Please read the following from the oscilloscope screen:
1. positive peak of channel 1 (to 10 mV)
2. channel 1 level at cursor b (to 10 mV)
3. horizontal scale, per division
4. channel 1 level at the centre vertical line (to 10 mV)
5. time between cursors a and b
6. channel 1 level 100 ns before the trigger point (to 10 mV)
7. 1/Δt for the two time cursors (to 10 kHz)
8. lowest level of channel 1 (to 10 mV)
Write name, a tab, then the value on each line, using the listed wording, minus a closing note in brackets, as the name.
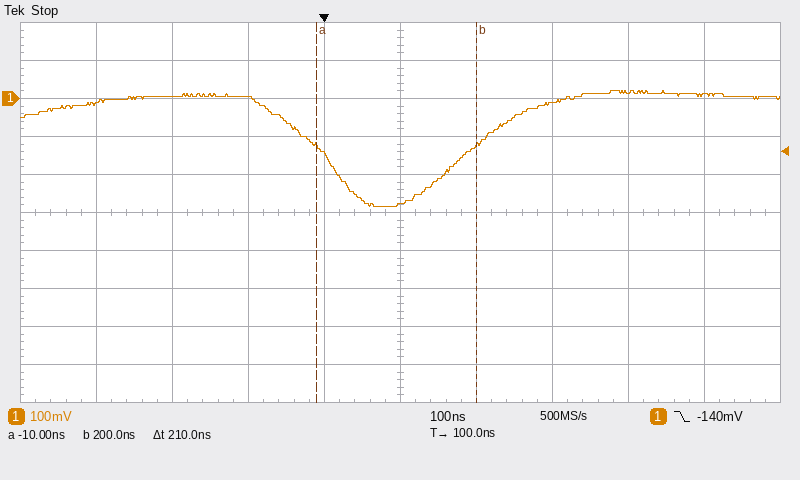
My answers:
positive peak of channel 1	20 mV
channel 1 level at cursor b	-120 mV
horizontal scale, per division	100 ns
channel 1 level at the centre vertical line	-280 mV
time between cursors a and b	210 ns
channel 1 level 100 ns before the trigger point	0 mV
1/Δt for the two time cursors	4.76 MHz
lowest level of channel 1	-280 mV
